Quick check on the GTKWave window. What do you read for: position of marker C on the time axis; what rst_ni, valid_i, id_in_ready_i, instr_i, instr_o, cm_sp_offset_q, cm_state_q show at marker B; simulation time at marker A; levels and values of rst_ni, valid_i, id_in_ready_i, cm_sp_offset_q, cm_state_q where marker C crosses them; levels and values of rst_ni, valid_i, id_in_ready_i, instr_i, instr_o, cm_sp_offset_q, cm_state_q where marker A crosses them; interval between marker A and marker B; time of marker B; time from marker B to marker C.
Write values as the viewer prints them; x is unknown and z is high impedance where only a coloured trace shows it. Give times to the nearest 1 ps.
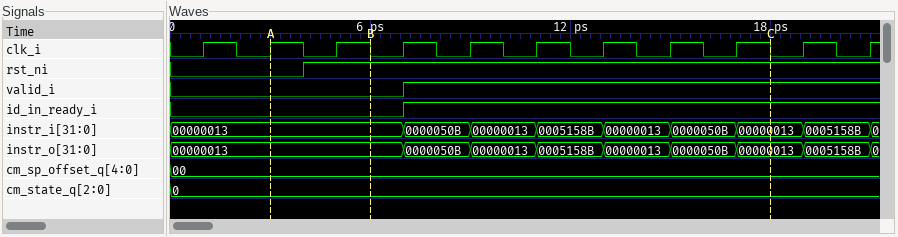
18 ps
rst_ni=1, valid_i=0, id_in_ready_i=0, instr_i=00000013, instr_o=00000013, cm_sp_offset_q=00, cm_state_q=0
3 ps
rst_ni=1, valid_i=1, id_in_ready_i=1, cm_sp_offset_q=00, cm_state_q=0
rst_ni=0, valid_i=0, id_in_ready_i=0, instr_i=00000013, instr_o=00000013, cm_sp_offset_q=00, cm_state_q=0
3 ps
6 ps
12 ps
